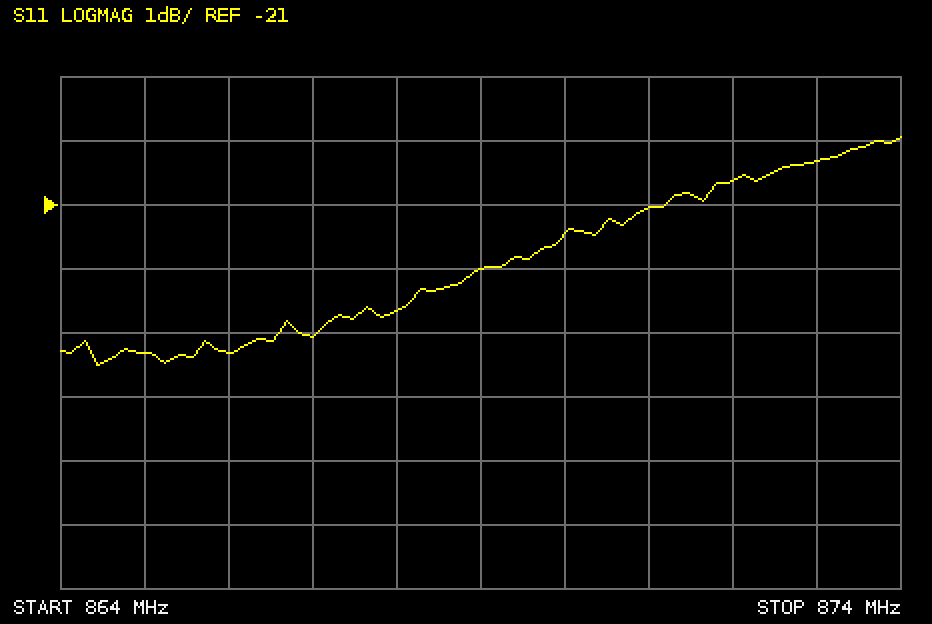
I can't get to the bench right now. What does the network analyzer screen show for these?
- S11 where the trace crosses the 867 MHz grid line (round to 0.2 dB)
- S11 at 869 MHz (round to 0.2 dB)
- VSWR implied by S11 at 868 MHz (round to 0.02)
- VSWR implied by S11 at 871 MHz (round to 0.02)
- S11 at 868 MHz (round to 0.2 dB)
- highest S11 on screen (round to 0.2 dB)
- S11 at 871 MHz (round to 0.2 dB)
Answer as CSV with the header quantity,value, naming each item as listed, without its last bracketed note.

quantity,value
S11 where the trace crosses the 867 MHz grid line,-23.0 dB
S11 at 869 MHz,-22.0 dB
VSWR implied by S11 at 868 MHz,1.16
VSWR implied by S11 at 871 MHz,1.20
S11 at 868 MHz,-22.6 dB
highest S11 on screen,-20.0 dB
S11 at 871 MHz,-21.0 dB
